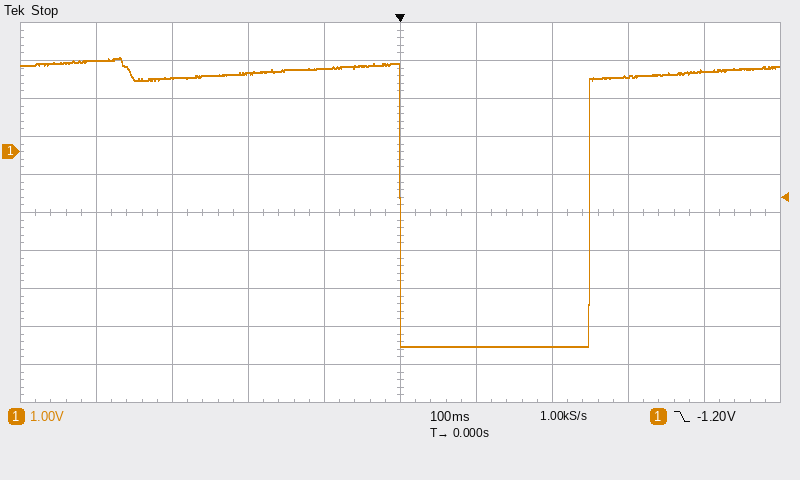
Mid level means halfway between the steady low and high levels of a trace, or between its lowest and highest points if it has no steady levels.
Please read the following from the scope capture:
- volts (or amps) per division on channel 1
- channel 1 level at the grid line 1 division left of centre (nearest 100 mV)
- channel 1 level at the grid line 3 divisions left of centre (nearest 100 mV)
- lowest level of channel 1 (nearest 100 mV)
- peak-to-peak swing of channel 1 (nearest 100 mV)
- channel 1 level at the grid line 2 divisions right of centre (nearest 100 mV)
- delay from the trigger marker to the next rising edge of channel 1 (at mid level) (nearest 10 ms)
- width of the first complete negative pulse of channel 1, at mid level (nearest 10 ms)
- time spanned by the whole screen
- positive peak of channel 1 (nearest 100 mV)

1 V
2.2 V
1.9 V
-5.1 V
7.6 V
-5.1 V
250 ms
250 ms
1 s
2.5 V
